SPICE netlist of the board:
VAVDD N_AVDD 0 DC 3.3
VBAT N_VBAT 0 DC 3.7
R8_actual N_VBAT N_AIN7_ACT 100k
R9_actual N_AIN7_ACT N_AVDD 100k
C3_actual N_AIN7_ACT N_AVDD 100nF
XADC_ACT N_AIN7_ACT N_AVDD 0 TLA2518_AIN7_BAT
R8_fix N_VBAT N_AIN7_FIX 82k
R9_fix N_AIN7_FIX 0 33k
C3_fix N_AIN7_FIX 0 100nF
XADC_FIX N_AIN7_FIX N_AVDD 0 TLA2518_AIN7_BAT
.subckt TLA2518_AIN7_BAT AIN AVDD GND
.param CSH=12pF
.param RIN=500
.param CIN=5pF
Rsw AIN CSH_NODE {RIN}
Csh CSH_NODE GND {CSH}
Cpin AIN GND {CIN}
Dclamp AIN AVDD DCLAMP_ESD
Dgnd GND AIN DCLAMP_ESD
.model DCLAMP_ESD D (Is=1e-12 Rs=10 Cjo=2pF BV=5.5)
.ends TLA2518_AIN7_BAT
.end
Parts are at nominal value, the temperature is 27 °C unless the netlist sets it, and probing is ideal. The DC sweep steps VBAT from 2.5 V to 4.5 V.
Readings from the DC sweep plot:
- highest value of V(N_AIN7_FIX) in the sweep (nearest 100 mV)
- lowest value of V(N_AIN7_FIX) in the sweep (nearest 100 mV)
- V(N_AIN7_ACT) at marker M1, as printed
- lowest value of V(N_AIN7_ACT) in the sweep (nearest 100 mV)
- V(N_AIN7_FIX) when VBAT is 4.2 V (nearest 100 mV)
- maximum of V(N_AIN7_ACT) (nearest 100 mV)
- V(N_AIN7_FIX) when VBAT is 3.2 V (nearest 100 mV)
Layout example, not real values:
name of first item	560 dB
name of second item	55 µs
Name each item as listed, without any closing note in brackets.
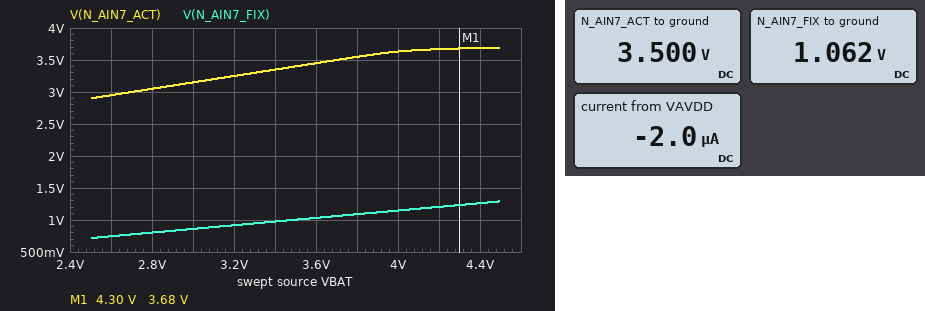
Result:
highest value of V(N_AIN7_FIX) in the sweep	1.3 V
lowest value of V(N_AIN7_FIX) in the sweep	700 mV
V(N_AIN7_ACT) at marker M1, as printed	3.68 V
lowest value of V(N_AIN7_ACT) in the sweep	2.9 V
V(N_AIN7_FIX) when VBAT is 4.2 V	1.2 V
maximum of V(N_AIN7_ACT)	3.7 V
V(N_AIN7_FIX) when VBAT is 3.2 V	900 mV
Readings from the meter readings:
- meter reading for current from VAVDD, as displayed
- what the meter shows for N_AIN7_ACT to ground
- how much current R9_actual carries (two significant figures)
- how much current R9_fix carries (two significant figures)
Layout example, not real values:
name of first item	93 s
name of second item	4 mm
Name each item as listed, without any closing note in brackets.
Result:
meter reading for current from VAVDD, as displayed	-2.0 µA
what the meter shows for N_AIN7_ACT to ground	3.500 V
how much current R9_actual carries	2.0 µA
how much current R9_fix carries	32 µA
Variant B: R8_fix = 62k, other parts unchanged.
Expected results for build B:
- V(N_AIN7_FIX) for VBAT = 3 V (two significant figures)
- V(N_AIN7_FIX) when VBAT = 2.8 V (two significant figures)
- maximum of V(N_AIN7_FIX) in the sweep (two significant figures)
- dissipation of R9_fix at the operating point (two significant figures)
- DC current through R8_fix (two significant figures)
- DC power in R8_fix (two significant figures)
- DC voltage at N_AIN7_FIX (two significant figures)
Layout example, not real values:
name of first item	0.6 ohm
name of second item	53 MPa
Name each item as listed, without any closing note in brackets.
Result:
V(N_AIN7_FIX) for VBAT = 3 V	1.0 V
V(N_AIN7_FIX) when VBAT = 2.8 V	970 mV
maximum of V(N_AIN7_FIX) in the sweep	1.6 V
dissipation of R9_fix at the operating point	50 µW
DC current through R8_fix	39 µA
DC power in R8_fix	94 µW
DC voltage at N_AIN7_FIX	1.3 V
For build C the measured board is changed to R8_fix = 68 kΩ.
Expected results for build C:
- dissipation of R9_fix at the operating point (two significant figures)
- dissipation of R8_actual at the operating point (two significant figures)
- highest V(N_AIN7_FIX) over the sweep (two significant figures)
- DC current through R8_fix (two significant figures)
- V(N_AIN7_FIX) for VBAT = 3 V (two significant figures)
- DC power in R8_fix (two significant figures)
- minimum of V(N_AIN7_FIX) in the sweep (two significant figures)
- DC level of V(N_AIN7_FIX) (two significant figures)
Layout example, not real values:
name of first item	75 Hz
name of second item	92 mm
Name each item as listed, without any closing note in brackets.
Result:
dissipation of R9_fix at the operating point	44 µW
dissipation of R8_actual at the operating point	400 nW
highest V(N_AIN7_FIX) over the sweep	1.5 V
DC current through R8_fix	37 µA
V(N_AIN7_FIX) for VBAT = 3 V	980 mV
DC power in R8_fix	91 µW
minimum of V(N_AIN7_FIX) in the sweep	820 mV
DC level of V(N_AIN7_FIX)	1.2 V
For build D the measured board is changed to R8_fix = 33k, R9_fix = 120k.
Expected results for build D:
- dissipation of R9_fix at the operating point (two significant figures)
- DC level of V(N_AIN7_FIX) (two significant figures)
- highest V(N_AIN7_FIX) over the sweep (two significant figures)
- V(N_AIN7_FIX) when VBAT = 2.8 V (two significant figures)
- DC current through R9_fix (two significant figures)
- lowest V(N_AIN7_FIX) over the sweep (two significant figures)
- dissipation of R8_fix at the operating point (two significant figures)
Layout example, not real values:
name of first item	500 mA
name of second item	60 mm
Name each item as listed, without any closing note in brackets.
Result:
dissipation of R9_fix at the operating point	70 µW
DC level of V(N_AIN7_FIX)	2.9 V
highest V(N_AIN7_FIX) over the sweep	3.5 V
V(N_AIN7_FIX) when VBAT = 2.8 V	2.2 V
DC current through R9_fix	24 µA
lowest V(N_AIN7_FIX) over the sweep	2.0 V
dissipation of R8_fix at the operating point	19 µW
